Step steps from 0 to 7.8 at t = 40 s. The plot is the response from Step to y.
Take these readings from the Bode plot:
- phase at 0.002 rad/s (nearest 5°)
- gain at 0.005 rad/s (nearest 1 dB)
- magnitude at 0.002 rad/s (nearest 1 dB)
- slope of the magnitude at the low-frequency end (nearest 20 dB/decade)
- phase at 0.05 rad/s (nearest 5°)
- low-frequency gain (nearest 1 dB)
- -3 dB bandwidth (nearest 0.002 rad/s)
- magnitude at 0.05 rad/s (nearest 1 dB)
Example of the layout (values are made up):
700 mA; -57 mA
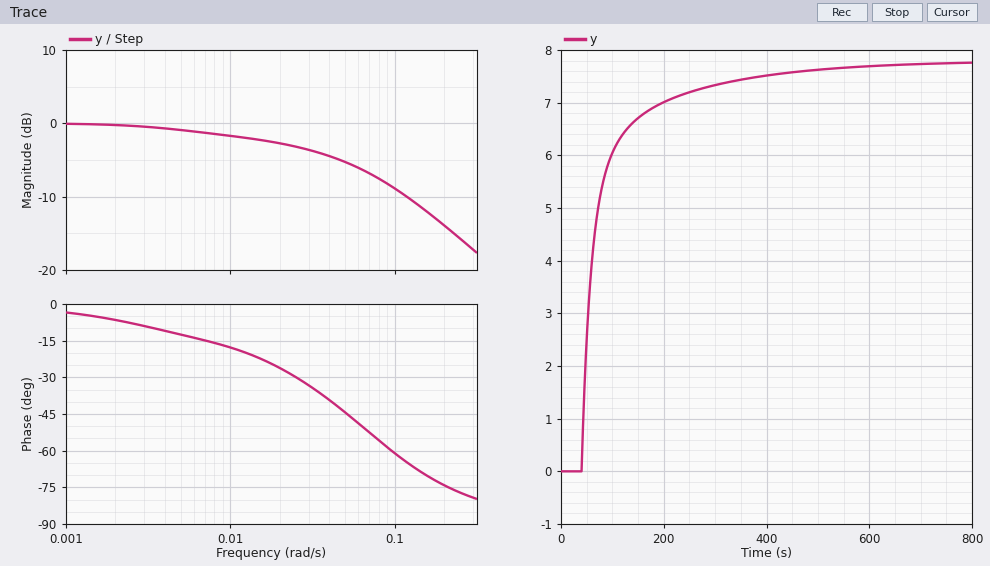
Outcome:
-5°; -1 dB; 0 dB; 0 dB/decade; -45°; 0 dB; 0.024 rad/s; -5 dB
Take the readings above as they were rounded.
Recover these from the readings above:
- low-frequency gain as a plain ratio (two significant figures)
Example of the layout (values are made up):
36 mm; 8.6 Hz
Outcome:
1.0
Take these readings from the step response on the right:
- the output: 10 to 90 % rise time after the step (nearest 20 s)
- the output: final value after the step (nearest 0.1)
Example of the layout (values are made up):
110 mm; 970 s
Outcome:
160 s; 7.8
